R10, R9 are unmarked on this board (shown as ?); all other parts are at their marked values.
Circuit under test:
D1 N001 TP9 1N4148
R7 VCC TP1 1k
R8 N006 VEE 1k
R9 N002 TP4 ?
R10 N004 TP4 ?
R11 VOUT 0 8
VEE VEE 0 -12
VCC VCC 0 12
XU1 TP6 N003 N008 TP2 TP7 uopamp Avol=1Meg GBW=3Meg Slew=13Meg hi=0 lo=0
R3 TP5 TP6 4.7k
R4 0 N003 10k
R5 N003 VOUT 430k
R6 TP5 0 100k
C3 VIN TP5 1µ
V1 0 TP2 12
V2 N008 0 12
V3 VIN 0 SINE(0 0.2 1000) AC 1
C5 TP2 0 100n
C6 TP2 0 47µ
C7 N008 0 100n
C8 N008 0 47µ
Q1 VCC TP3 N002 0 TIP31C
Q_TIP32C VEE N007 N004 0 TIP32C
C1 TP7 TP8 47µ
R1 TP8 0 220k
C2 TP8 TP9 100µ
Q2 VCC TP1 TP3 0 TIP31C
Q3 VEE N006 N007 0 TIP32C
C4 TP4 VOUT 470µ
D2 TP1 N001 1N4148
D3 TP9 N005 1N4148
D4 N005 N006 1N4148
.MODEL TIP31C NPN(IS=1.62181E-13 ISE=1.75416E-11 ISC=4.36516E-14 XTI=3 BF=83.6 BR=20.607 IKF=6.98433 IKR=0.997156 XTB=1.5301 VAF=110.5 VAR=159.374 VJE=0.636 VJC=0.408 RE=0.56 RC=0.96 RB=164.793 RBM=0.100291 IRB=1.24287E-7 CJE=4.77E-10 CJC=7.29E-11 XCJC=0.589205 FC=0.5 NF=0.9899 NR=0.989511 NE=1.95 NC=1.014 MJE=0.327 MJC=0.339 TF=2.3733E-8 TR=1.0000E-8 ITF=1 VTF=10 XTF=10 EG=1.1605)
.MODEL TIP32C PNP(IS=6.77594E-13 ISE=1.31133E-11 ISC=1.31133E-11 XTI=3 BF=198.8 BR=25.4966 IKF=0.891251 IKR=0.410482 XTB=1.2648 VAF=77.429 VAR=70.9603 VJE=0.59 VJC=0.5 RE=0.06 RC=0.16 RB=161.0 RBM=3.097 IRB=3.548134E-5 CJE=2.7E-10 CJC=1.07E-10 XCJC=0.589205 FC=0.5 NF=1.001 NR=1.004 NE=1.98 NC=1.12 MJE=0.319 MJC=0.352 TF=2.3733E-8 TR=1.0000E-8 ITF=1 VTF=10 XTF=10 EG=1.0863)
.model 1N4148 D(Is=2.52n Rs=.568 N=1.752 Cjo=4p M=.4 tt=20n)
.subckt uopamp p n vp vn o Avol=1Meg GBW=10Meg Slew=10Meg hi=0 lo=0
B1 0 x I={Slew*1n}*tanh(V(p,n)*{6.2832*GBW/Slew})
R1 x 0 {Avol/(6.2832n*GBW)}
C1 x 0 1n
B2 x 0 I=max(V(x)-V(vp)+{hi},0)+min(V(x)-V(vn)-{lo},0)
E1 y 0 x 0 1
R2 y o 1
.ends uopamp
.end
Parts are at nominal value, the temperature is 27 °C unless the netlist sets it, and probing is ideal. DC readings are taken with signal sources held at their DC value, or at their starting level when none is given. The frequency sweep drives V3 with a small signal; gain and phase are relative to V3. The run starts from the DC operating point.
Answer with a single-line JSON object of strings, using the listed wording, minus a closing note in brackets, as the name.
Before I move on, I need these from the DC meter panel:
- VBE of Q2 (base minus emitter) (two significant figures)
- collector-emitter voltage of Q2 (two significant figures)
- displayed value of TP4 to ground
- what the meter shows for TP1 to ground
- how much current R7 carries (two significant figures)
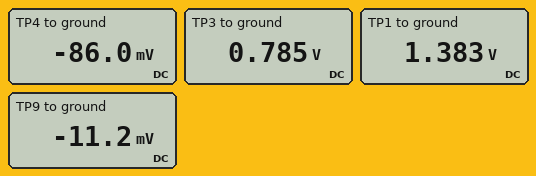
{"VBE of Q2 (base minus emitter)": "600 mV", "collector-emitter voltage of Q2": "11 V", "displayed value of TP4 to ground": "-86.0 mV", "what the meter shows for TP1 to ground": "1.383 V", "how much current R7 carries": "11 mA"}
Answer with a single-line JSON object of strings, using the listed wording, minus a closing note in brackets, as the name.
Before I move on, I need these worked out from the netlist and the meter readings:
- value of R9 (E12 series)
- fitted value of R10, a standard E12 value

{"value of R9": "0.18 Ω", "fitted value of R10, a standard E12 value": "0.22 Ω"}
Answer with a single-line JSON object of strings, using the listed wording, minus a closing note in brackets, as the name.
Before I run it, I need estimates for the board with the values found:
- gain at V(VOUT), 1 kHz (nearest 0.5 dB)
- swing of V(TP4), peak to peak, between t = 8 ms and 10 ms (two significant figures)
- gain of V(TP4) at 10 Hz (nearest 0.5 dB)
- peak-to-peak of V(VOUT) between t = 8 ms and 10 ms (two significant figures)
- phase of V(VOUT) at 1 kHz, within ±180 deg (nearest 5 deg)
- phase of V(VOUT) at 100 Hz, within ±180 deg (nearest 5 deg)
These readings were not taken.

{"gain at V(VOUT), 1 kHz": "33.0 dB", "swing of V(TP4), peak to peak, between t = 8 ms and 10 ms": "18 V", "gain of V(TP4) at 10 Hz": "45.5 dB", "peak-to-peak of V(VOUT) between t = 8 ms and 10 ms": "18 V", "phase of V(VOUT) at 1 kHz, within ±180 deg": "0 deg", "phase of V(VOUT) at 100 Hz, within ±180 deg": "0 deg"}
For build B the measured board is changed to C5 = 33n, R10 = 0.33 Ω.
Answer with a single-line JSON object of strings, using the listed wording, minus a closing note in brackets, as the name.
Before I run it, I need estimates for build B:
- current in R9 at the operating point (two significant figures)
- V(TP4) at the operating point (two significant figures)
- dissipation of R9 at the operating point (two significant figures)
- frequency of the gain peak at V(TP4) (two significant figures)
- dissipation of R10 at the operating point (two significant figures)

{"current in R9 at the operating point": "200 mA", "V(TP4) at the operating point": "-72 mV", "dissipation of R9 at the operating point": "7.1 mW", "frequency of the gain peak at V(TP4)": "140 mHz", "dissipation of R10 at the operating point": "13 mW"}
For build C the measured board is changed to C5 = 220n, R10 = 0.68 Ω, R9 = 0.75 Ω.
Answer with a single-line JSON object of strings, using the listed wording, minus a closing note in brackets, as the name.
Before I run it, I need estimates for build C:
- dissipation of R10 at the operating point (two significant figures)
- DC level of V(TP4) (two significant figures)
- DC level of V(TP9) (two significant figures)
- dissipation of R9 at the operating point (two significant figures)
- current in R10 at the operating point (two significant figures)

{"dissipation of R10 at the operating point": "12 mW", "DC level of V(TP4)": "-76 mV", "DC level of V(TP9)": "-7.3 mV", "dissipation of R9 at the operating point": "13 mW", "current in R10 at the operating point": "130 mA"}
